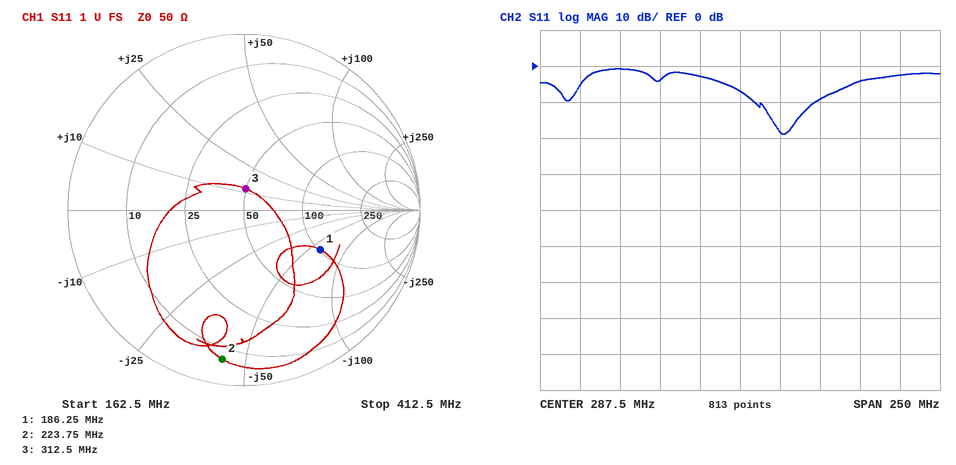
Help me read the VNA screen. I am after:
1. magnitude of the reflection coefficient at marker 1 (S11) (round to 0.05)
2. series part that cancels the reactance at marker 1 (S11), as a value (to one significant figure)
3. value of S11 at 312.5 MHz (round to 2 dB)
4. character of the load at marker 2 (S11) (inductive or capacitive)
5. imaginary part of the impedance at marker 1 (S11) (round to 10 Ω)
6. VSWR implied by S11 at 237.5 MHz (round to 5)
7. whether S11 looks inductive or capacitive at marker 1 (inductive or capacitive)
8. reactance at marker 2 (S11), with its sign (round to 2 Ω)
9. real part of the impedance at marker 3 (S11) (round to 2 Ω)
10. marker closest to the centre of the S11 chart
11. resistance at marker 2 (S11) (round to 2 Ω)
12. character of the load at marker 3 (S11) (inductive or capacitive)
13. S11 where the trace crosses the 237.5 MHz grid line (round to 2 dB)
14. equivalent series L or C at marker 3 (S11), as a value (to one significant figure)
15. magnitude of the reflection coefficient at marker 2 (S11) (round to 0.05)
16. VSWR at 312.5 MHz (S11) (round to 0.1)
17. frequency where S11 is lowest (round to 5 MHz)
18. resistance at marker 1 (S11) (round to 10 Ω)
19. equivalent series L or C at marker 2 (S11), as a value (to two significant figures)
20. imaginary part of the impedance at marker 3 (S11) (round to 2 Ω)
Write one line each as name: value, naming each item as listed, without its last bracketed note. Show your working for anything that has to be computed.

magnitude of the reflection coefficient at marker 1 (S11): 0.50
series part that cancels the reactance at marker 1 (S11), as a value: L = 60 Ω/(2π × 186.25 MHz) ≈ 51.3 nH, so 50 nH to one significant figure
value of S11 at 312.5 MHz: -18 dB
character of the load at marker 2 (S11): capacitive
imaginary part of the impedance at marker 1 (S11): -60 Ω
VSWR implied by S11 at 237.5 MHz: |Γ| = 10^(-4/20) = 0.6310; VSWR = (1 + 0.6310)/(1 − 0.6310) ≈ 4.42, so 5 to the nearest 5
whether S11 looks inductive or capacitive at marker 1: capacitive
reactance at marker 2 (S11), with its sign: -42 Ω
real part of the impedance at marker 3 (S11): 50 Ω
marker closest to the centre of the S11 chart: marker 3
resistance at marker 2 (S11): 6 Ω
character of the load at marker 3 (S11): inductive
S11 where the trace crosses the 237.5 MHz grid line: -4 dB
equivalent series L or C at marker 3 (S11), as a value: L = 12 Ω/(2π × 312.5 MHz) ≈ 6 nH
magnitude of the reflection coefficient at marker 2 (S11): 0.85
VSWR at 312.5 MHz (S11): |Γ| = 10^(-18/20) = 0.1259; VSWR = (1 + 0.1259)/(1 − 0.1259) ≈ 1.3
frequency where S11 is lowest: 315 MHz
resistance at marker 1 (S11): 100 Ω
equivalent series L or C at marker 2 (S11), as a value: C = 1/(2π × 223.75 MHz × 42 Ω) ≈ 17 pF
imaginary part of the impedance at marker 3 (S11): +12 Ω
